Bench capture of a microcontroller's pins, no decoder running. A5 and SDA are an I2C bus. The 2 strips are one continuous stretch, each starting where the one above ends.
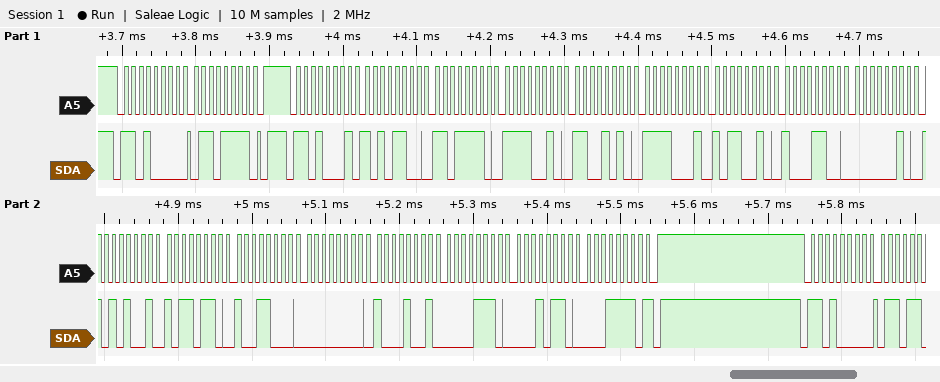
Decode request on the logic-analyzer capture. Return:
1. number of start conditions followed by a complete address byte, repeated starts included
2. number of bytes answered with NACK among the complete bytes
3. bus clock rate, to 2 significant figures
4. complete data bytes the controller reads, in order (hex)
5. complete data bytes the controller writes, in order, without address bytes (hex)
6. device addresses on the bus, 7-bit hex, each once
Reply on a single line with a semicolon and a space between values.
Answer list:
3; 1; 100 kHz; AC DE F2 CA F1 B2 8C 02 A9 B6 98 00 89 0E 16 1E; 6F; 0x68
